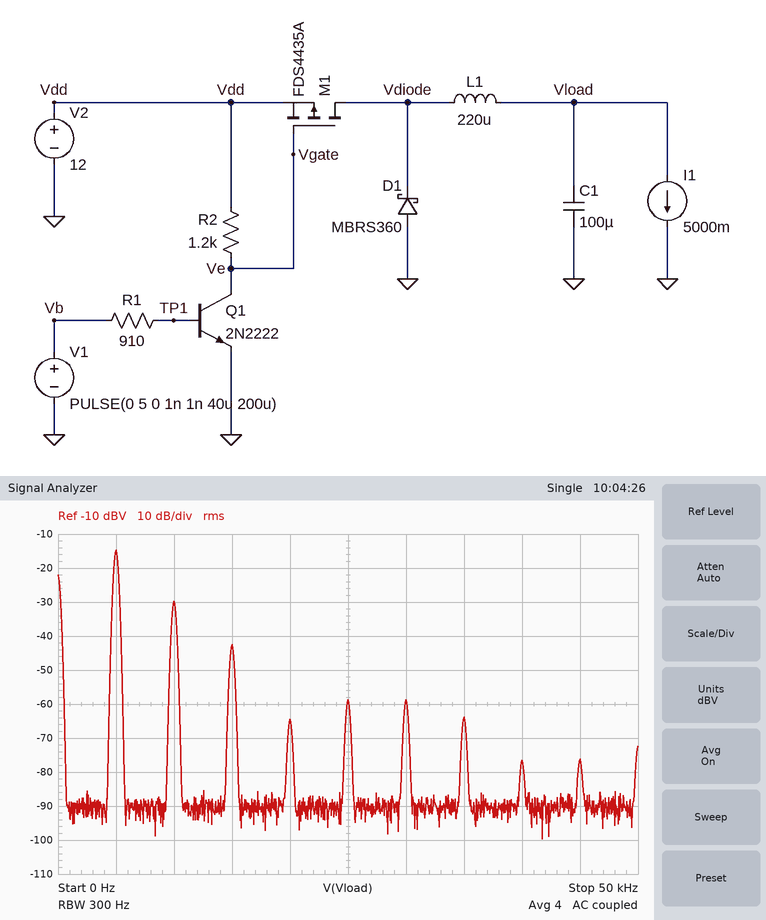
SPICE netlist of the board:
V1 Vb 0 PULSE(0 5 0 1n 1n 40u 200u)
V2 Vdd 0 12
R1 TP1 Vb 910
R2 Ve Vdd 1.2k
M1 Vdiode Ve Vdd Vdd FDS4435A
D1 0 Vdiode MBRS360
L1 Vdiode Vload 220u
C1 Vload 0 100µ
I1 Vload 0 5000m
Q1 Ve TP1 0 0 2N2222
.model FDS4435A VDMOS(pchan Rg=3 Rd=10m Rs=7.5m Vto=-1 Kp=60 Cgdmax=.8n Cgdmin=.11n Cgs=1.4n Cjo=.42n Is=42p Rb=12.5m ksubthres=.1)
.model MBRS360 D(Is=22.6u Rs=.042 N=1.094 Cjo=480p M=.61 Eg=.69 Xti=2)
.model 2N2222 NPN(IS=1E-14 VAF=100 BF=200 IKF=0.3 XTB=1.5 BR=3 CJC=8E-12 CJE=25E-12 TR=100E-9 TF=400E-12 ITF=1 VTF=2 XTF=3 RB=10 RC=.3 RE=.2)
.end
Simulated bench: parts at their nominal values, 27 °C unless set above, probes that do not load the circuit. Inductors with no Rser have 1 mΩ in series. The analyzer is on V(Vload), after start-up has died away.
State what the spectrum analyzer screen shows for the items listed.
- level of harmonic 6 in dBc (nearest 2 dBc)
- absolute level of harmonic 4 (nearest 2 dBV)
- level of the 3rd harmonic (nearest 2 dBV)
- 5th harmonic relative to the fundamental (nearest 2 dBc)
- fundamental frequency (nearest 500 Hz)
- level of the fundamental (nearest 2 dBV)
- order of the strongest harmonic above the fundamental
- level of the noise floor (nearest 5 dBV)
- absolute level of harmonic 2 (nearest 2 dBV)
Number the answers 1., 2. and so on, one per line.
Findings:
1. -44 dBc
2. -64 dBV
3. -42 dBV
4. -44 dBc
5. 5.0 kHz
6. -14 dBV
7. 2
8. -90 dBV
9. -30 dBV
